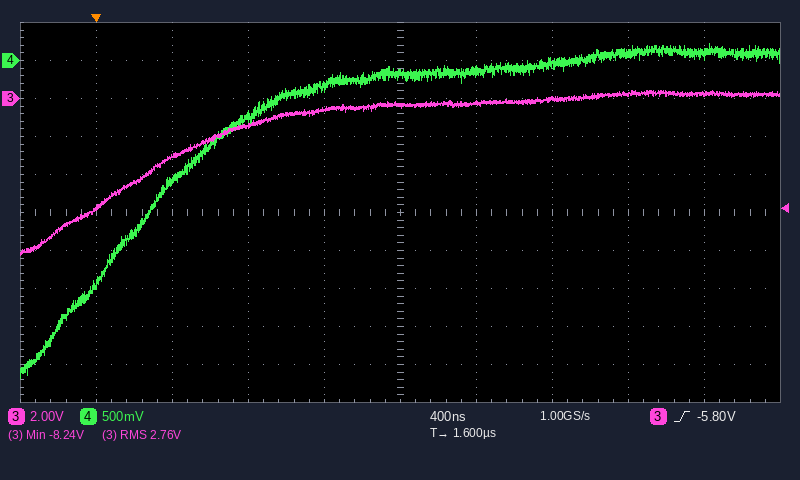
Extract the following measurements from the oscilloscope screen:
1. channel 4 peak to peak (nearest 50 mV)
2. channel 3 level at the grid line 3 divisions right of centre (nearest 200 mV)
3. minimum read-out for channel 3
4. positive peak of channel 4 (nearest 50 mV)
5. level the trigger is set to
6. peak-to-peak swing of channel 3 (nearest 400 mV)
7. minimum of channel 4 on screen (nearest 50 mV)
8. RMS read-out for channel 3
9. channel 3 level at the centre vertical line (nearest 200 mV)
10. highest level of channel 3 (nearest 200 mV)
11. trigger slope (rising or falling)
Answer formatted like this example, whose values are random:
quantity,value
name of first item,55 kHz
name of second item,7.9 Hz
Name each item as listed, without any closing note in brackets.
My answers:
quantity,value
channel 4 peak to peak,4.40 V
channel 3 level at the grid line 3 divisions right of centre,200 mV
minimum read-out for channel 3,-8.24 V
positive peak of channel 4,200 mV
level the trigger is set to,-5.80 V
peak-to-peak swing of channel 3,8.8 V
minimum of channel 4 on screen,-4.20 V
RMS read-out for channel 3,2.76 V
channel 3 level at the centre vertical line,-400 mV
highest level of channel 3,400 mV
trigger slope,rising
